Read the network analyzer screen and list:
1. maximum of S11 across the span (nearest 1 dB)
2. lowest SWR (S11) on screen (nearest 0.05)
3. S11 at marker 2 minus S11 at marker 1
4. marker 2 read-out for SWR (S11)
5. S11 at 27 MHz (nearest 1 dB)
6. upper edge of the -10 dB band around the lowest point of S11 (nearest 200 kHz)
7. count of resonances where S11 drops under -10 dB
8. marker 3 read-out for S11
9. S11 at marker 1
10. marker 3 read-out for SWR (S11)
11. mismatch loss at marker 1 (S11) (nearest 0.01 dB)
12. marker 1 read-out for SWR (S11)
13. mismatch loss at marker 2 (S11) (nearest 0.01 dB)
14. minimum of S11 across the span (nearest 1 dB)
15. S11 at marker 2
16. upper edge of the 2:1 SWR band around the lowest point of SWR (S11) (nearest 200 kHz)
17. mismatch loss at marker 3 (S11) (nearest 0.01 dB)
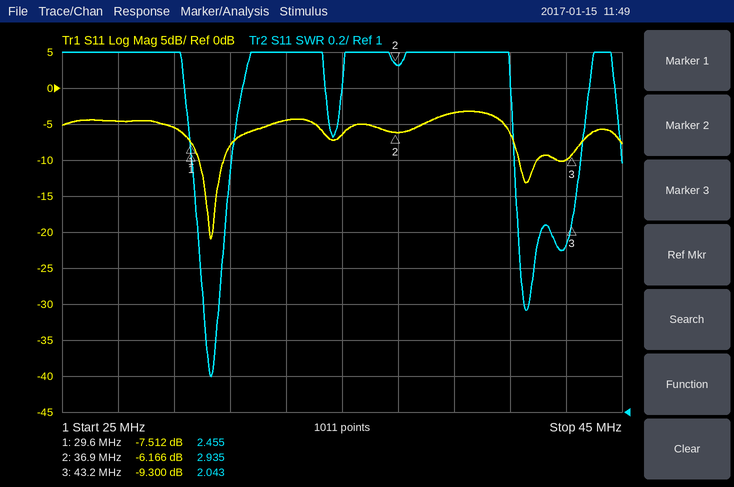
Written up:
-3 dB
1.20
1.346 dB
2.935
-5 dB
30.8 MHz
2
-9.300 dB
-7.512 dB
2.043
0.85 dB
2.455
1.20 dB
-21 dB
-6.166 dB
30.8 MHz
0.54 dB
